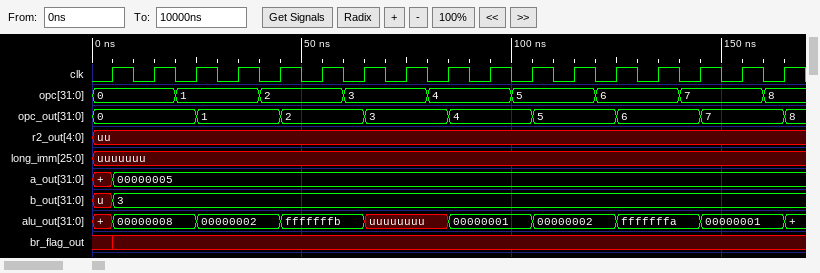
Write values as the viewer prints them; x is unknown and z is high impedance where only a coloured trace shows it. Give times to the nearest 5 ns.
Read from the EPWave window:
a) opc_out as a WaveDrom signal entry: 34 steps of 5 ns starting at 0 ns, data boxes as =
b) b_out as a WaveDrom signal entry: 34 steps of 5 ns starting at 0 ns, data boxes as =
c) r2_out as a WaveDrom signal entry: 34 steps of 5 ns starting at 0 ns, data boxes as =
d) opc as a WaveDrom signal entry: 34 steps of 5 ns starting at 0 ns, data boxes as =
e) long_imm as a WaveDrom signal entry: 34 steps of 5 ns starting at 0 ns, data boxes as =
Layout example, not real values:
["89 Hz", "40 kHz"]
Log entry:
["{name: 'opc_out', wave: '=....=...=...=...=...=...=...=...=', data: '0 1 2 3 4 5 6 7 8'}", "{name: 'b_out', wave: 'x=................................', data: '3'}", "{name: 'r2_out', wave: 'x.................................'}", "{name: 'opc', wave: '=...=...=...=...=...=...=...=...=.', data: '0 1 2 3 4 5 6 7 8'}", "{name: 'long_imm', wave: 'x.................................'}"]
